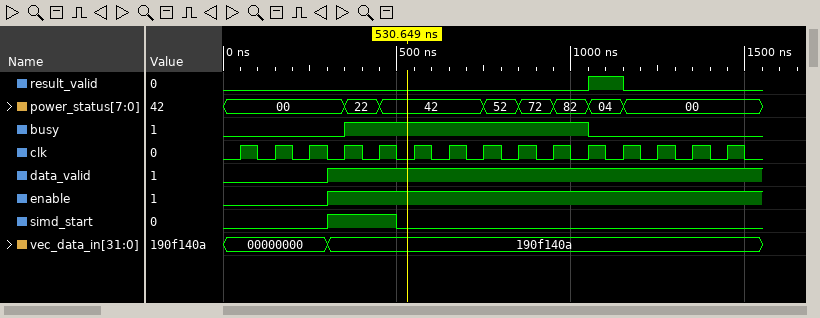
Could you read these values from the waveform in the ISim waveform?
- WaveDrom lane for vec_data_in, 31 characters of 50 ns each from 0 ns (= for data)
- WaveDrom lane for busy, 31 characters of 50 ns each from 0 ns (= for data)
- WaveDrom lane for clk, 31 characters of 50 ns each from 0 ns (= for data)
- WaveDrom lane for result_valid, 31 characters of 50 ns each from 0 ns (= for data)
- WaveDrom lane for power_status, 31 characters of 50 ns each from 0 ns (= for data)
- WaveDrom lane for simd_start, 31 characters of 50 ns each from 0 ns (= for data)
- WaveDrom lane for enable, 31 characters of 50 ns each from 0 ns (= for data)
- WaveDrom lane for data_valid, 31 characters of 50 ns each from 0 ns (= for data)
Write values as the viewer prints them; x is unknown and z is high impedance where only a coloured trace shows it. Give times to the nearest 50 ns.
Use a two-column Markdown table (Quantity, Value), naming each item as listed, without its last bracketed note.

| Quantity | Value |
|---|---|
| WaveDrom lane for vec_data_in, 31 characters of 50 ns each from 0 ns | {name: 'vec_data_in', wave: '=.....=........................', data: '00000000 190f140a'} |
| WaveDrom lane for busy, 31 characters of 50 ns each from 0 ns | {name: 'busy', wave: '0......1.............0.........'} |
| WaveDrom lane for clk, 31 characters of 50 ns each from 0 ns | {name: 'clk', wave: '0101010101010101010101010101010'} |
| WaveDrom lane for result_valid, 31 characters of 50 ns each from 0 ns | {name: 'result_valid', wave: '0....................1.0.......'} |
| WaveDrom lane for power_status, 31 characters of 50 ns each from 0 ns | {name: 'power_status', wave: '=......=.=.....=.=.=.=.=.......', data: '00 22 42 52 72 82 04 00'} |
| WaveDrom lane for simd_start, 31 characters of 50 ns each from 0 ns | {name: 'simd_start', wave: '0.....1...0....................'} |
| WaveDrom lane for enable, 31 characters of 50 ns each from 0 ns | {name: 'enable', wave: '0.....1........................'} |
| WaveDrom lane for data_valid, 31 characters of 50 ns each from 0 ns | {name: 'data_valid', wave: '0.....1........................'} |
